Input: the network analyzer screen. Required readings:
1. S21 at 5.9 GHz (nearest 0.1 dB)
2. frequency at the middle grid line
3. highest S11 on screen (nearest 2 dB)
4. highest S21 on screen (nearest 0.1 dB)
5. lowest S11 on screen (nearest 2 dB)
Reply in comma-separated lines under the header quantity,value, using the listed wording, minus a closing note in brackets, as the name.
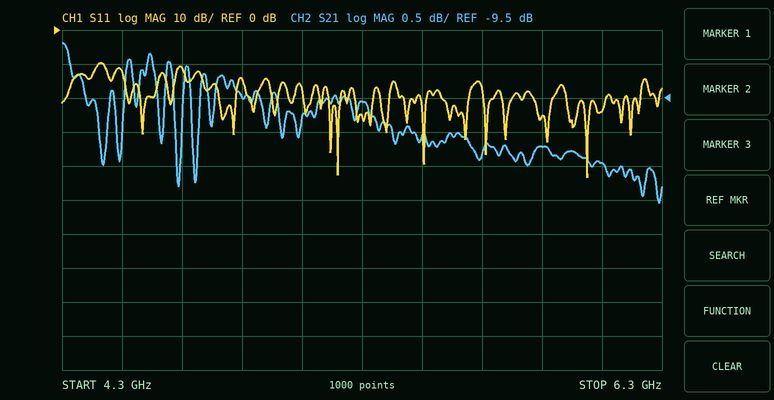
quantity,value
S21 at 5.9 GHz,-10.2 dB
frequency at the middle grid line,5.3 GHz
highest S11 on screen,-10 dB
highest S21 on screen,-8.7 dB
lowest S11 on screen,-44 dB
